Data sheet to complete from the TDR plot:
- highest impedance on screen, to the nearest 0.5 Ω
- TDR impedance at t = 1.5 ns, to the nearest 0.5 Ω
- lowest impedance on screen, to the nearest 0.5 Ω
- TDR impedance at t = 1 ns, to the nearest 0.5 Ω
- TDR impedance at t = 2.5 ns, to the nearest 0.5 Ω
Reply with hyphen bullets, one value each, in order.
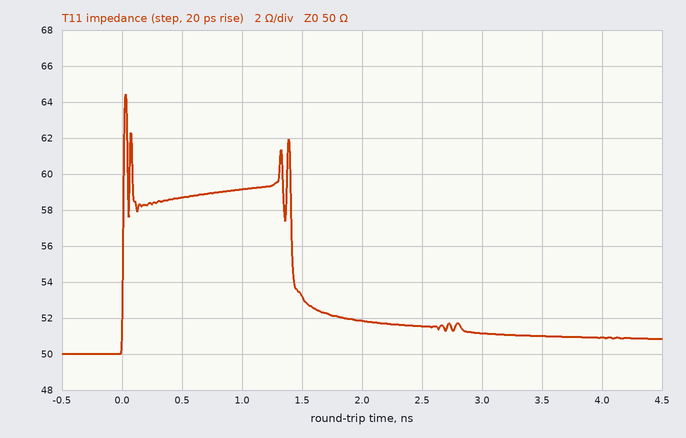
- 64.5 Ω
- 53.0 Ω
- 50.0 Ω
- 59.0 Ω
- 51.5 Ω
